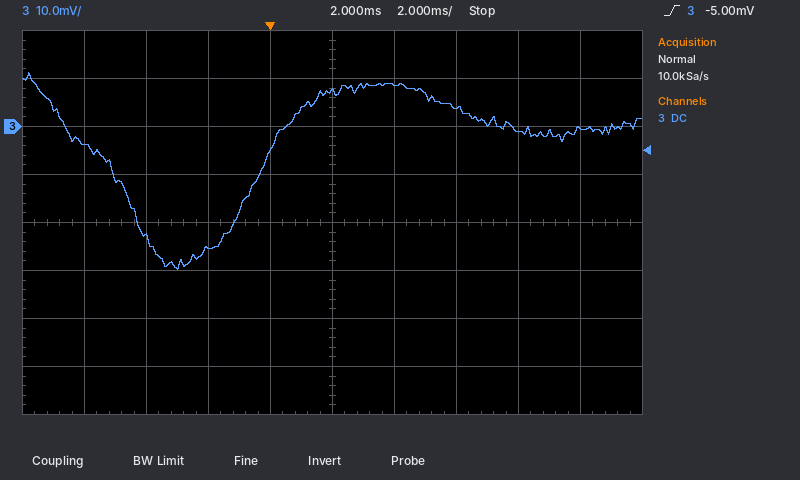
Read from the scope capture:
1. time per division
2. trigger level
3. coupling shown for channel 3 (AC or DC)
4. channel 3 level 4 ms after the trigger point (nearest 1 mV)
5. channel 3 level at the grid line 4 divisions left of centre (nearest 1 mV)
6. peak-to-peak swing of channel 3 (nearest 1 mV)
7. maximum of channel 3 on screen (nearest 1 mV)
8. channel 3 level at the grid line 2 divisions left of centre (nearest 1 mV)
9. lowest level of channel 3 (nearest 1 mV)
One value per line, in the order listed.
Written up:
2 ms
-5.00 mV
DC
9 mV
-4 mV
41 mV
11 mV
-25 mV
-30 mV
